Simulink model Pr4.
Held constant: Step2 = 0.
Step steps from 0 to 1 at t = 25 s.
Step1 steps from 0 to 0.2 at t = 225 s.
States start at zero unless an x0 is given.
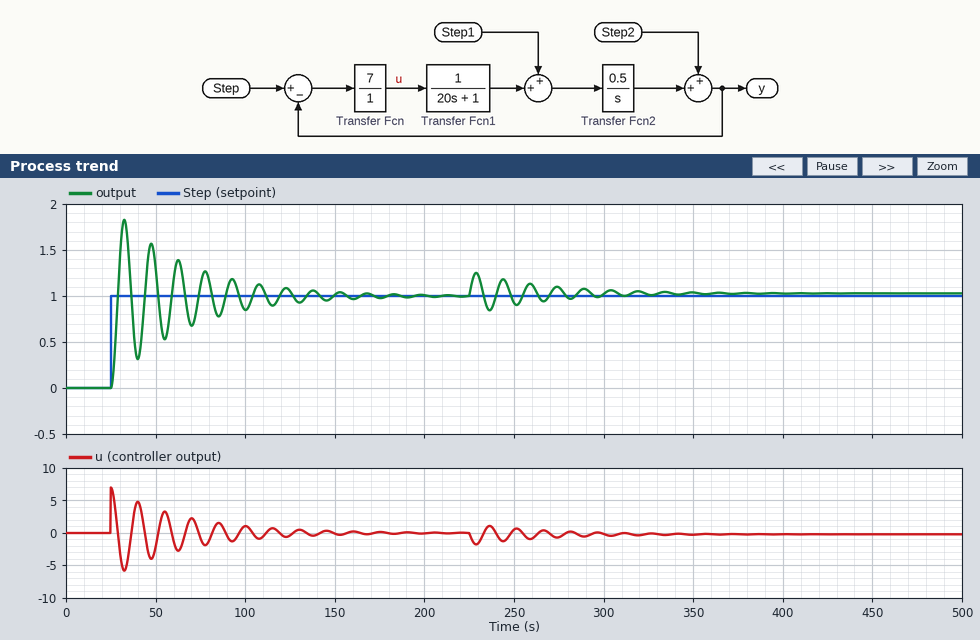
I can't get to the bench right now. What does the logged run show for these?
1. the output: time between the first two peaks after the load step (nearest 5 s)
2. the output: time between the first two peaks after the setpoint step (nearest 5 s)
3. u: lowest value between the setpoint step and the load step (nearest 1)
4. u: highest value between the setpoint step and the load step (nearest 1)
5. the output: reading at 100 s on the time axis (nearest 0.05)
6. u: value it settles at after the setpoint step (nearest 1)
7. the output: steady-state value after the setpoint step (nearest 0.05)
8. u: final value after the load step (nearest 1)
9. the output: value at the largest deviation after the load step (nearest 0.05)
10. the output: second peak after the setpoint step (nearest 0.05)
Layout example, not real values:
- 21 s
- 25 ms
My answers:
- 15 s
- 15 s
- -6
- 7
- 0.85
- 0
- 1.00
- 0
- 1.25
- 1.55
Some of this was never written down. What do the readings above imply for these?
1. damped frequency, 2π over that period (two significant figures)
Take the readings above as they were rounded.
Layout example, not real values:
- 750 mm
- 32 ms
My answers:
- 0.42 rad/s
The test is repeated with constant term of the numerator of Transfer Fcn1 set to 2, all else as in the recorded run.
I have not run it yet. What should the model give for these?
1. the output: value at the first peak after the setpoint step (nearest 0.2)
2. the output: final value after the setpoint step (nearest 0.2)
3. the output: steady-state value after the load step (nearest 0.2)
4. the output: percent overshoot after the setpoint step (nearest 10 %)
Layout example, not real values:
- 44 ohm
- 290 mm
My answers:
- 1.8
- 1.0
- 1.0
- 90 %
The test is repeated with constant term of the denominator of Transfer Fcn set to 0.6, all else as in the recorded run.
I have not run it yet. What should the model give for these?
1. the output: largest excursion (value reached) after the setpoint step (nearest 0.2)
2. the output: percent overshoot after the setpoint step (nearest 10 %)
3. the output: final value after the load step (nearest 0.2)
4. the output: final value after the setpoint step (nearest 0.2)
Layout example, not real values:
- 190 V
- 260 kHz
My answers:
- 1.8
- 90 %
- 1.0
- 1.0
